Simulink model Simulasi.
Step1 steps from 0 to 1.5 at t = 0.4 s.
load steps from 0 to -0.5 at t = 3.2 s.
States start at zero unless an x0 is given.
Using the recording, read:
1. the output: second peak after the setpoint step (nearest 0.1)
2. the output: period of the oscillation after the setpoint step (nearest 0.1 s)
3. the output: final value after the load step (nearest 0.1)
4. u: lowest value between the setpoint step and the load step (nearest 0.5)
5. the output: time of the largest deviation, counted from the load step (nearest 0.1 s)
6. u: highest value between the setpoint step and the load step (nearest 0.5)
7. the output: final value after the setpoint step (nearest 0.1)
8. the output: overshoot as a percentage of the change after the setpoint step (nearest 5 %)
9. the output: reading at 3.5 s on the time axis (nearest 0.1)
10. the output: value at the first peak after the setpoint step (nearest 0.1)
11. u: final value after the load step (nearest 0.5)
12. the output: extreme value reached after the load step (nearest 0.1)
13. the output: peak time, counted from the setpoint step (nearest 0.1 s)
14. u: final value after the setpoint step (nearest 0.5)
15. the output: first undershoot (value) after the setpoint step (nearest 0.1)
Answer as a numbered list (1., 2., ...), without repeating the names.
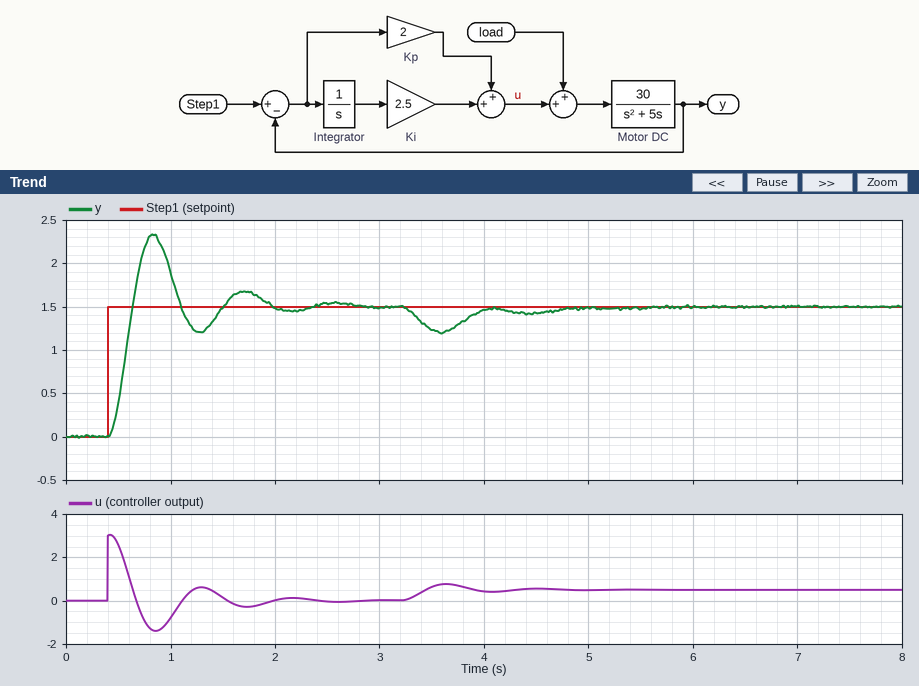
1. 1.7
2. 0.9 s
3. 1.5
4. -1.5
5. 0.4 s
6. 3.0
7. 1.5
8. 55 %
9. 1.2
10. 2.3
11. 0.5
12. 1.2
13. 0.4 s
14. 0.0
15. 1.2
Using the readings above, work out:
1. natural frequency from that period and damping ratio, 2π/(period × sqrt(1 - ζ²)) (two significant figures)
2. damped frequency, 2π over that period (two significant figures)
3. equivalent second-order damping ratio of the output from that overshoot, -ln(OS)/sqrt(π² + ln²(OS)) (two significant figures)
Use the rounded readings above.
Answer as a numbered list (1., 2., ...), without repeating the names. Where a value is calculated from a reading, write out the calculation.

1. 2π / (0.9 × sqrt(1 - 0.19²)) = 7.1 rad/s
2. 2π / 0.9 = 7.0 rad/s
3. ln(0.55) = -0.598; 0.598 / sqrt(9.870 + 0.357) = 0.19
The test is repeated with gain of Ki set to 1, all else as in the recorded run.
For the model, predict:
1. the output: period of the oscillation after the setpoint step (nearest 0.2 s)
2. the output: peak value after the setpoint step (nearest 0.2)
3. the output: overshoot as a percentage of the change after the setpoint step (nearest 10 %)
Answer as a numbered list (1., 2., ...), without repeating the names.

1. 0.8 s
2. 2.2
3. 40 %
